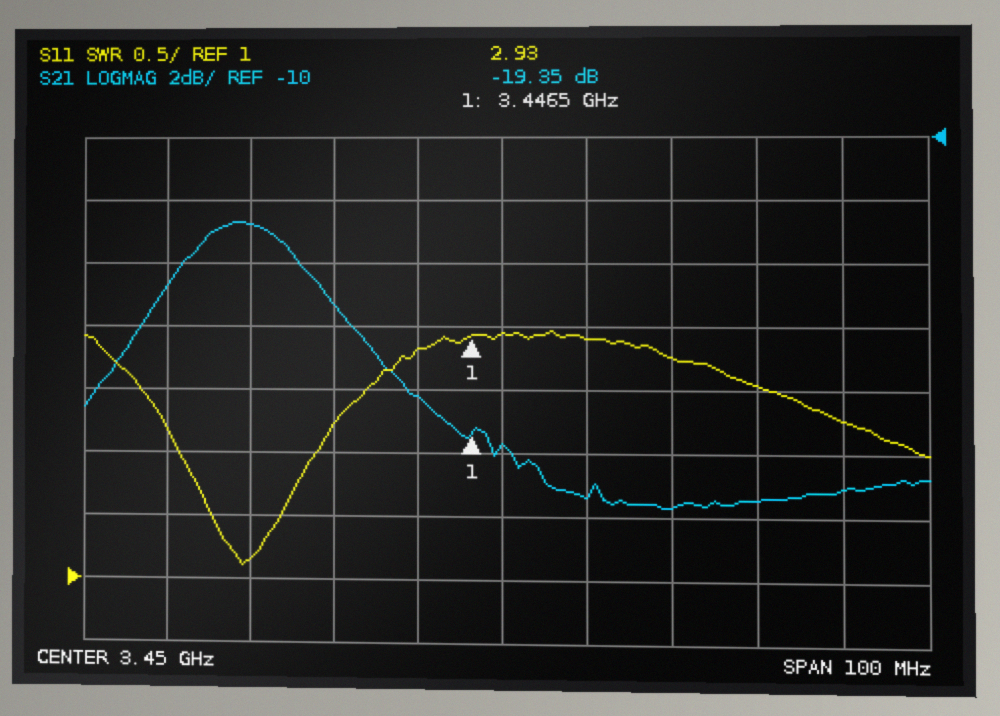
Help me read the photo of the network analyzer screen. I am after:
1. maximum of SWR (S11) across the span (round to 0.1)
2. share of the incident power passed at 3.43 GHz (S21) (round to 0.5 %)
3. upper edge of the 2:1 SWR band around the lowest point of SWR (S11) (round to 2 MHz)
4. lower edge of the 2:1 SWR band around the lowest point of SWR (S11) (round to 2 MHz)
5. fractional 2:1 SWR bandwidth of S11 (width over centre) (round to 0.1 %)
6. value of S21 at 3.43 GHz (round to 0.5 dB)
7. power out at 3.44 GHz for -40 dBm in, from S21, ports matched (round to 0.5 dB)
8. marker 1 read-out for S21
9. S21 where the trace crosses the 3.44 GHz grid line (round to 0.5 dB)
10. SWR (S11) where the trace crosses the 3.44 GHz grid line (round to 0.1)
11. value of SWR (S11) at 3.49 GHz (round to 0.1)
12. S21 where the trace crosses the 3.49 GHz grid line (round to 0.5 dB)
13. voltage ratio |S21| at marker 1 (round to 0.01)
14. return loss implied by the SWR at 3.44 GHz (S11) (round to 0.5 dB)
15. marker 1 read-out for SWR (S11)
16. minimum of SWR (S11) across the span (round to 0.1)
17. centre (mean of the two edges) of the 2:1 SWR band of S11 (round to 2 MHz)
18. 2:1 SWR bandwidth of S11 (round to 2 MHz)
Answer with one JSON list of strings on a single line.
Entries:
["3.0", "3.0 %", "3.428 GHz", "3.412 GHz", "0.5 %", "-15.5 dB", "-58.0 dBm", "-19.35 dB", "-18.0 dB", "2.8", "2.3", "-21.0 dB", "0.11", "6.5 dB", "2.93", "1.1", "3.420 GHz", "16 MHz"]
